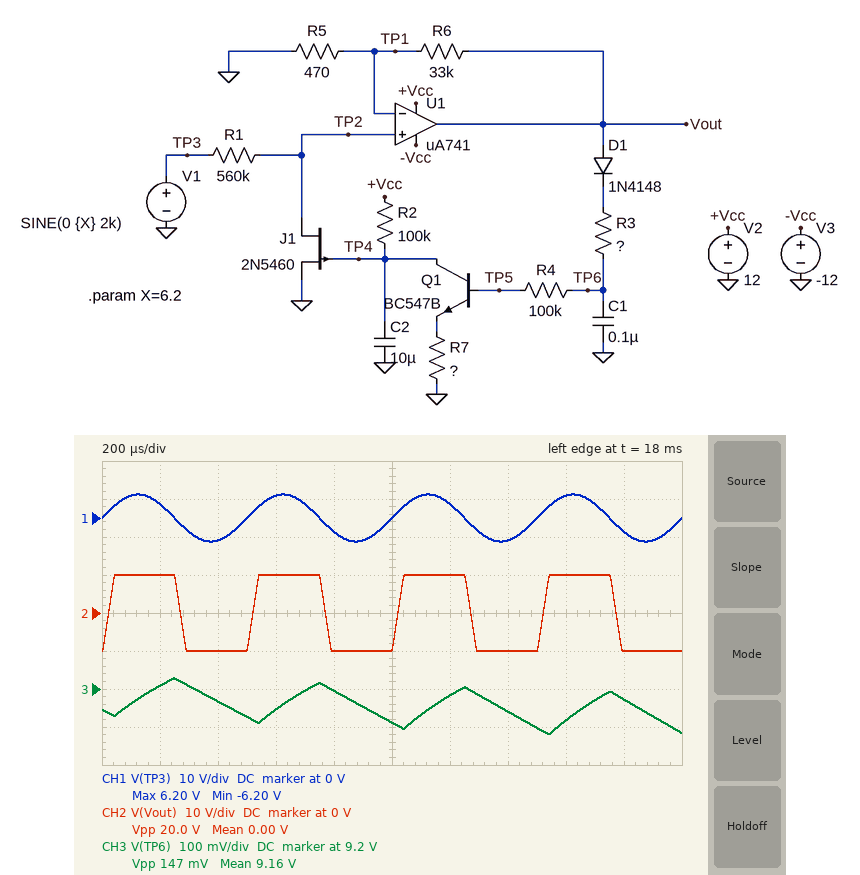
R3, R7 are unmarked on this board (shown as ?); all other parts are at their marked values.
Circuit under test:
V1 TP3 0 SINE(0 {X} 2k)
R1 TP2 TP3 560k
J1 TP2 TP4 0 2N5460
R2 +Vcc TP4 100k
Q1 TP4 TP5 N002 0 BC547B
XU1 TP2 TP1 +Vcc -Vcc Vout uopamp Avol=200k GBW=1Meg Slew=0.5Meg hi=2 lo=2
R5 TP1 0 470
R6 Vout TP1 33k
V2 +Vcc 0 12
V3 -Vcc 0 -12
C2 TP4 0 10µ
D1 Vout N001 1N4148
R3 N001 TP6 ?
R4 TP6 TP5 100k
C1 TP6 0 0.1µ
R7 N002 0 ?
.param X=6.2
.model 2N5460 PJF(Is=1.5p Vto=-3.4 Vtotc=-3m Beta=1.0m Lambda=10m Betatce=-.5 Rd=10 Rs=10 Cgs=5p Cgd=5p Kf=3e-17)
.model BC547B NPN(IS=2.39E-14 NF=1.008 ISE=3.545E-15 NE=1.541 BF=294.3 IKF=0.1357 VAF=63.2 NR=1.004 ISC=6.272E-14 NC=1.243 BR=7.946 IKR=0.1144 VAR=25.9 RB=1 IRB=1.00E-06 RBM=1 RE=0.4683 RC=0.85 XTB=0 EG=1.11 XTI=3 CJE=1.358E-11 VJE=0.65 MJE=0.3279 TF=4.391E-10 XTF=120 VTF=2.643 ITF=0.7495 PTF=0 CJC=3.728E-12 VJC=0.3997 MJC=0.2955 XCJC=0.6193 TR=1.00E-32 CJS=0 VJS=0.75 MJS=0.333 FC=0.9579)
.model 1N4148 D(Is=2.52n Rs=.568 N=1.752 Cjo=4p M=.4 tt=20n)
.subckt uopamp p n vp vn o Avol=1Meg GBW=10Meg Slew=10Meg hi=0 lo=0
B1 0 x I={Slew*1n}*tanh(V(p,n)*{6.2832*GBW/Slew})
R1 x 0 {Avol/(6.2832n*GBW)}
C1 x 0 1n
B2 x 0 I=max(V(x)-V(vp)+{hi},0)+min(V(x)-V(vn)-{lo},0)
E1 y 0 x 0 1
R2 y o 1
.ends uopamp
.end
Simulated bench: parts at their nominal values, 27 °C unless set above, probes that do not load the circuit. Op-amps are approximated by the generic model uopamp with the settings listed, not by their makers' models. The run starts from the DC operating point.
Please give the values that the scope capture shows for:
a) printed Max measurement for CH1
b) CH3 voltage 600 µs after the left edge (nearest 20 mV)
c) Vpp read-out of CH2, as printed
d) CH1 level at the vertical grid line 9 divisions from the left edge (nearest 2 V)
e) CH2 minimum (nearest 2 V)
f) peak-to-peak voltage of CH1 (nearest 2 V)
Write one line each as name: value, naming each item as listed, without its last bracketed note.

printed Max measurement for CH1: 6.20 V
CH3 voltage 600 µs after the left edge: 9.14 V
Vpp read-out of CH2, as printed: 20.0 V
CH1 level at the vertical grid line 9 divisions from the left edge: -4 V
CH2 minimum: -10 V
peak-to-peak voltage of CH1: 12 V
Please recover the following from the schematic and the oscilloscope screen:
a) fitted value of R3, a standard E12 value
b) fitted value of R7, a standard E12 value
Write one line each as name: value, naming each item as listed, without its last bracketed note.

fitted value of R3, a standard E12 value: 3.9 kΩ
fitted value of R7, a standard E12 value: 1.5 kΩ
